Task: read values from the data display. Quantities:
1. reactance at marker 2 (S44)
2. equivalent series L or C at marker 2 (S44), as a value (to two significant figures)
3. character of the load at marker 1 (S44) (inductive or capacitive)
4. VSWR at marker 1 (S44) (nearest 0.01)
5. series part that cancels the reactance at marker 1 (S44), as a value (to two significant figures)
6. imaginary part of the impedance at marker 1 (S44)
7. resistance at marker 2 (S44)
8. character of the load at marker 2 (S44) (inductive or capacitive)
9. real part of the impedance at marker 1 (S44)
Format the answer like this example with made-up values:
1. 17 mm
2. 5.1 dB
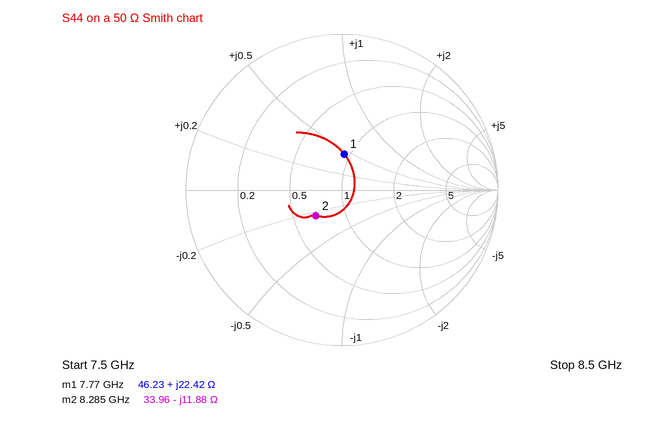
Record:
1. -11.88 Ω
2. 1.6 pF
3. inductive
4. 1.60
5. 910 fF
6. +22.42 Ω
7. 33.96 Ω
8. capacitive
9. 46.23 Ω
